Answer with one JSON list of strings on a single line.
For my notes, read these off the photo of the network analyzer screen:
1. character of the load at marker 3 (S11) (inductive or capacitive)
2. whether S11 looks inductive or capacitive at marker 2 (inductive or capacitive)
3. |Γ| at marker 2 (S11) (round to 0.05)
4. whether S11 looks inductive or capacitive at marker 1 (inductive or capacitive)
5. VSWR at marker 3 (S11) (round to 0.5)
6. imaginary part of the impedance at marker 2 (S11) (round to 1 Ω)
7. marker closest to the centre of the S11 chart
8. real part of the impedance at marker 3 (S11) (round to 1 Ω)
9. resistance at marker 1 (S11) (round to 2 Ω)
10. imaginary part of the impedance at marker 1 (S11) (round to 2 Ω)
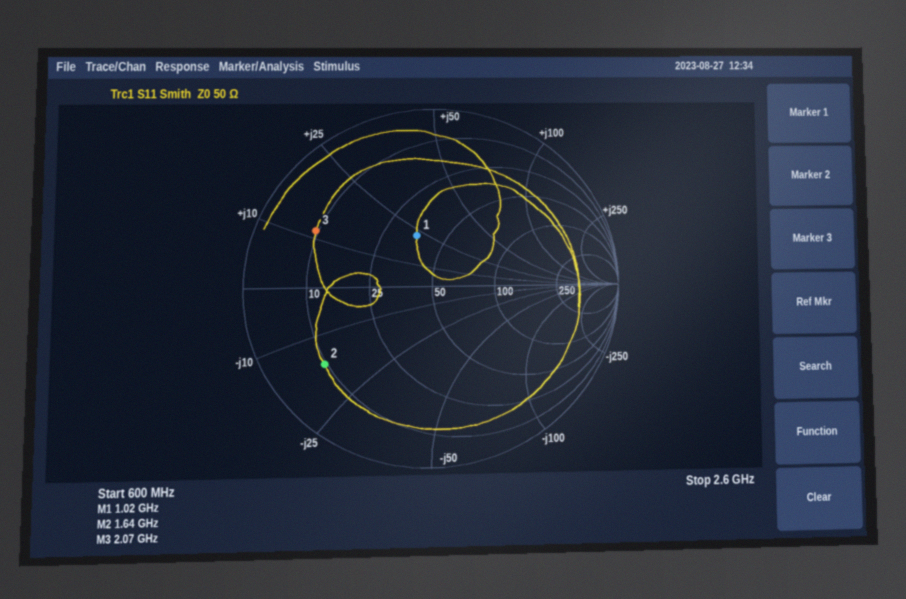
["inductive", "capacitive", "0.70", "inductive", "5.5", "-16 Ω", "marker 1", "9 Ω", "36 Ω", "+22 Ω"]
